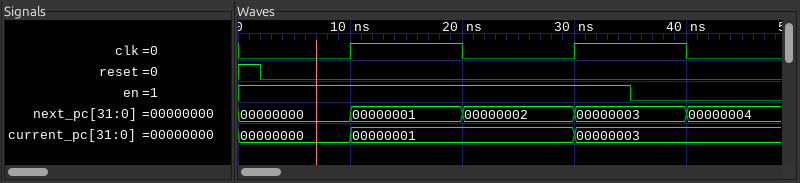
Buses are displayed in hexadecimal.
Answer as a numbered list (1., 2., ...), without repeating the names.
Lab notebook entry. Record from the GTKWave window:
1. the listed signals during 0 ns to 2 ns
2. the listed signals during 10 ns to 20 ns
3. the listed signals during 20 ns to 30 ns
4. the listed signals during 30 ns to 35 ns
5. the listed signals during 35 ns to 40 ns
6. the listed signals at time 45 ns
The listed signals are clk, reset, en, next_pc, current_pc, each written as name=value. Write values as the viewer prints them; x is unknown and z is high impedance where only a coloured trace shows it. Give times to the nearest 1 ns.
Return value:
1. clk=0, reset=1, en=1, next_pc=00000000, current_pc=00000000
2. clk=1, reset=0, en=1, next_pc=00000001, current_pc=00000001
3. clk=0, reset=0, en=1, next_pc=00000002, current_pc=00000001
4. clk=1, reset=0, en=1, next_pc=00000003, current_pc=00000003
5. clk=1, reset=0, en=0, next_pc=00000003, current_pc=00000003
6. clk=0, reset=0, en=0, next_pc=00000004, current_pc=00000003
